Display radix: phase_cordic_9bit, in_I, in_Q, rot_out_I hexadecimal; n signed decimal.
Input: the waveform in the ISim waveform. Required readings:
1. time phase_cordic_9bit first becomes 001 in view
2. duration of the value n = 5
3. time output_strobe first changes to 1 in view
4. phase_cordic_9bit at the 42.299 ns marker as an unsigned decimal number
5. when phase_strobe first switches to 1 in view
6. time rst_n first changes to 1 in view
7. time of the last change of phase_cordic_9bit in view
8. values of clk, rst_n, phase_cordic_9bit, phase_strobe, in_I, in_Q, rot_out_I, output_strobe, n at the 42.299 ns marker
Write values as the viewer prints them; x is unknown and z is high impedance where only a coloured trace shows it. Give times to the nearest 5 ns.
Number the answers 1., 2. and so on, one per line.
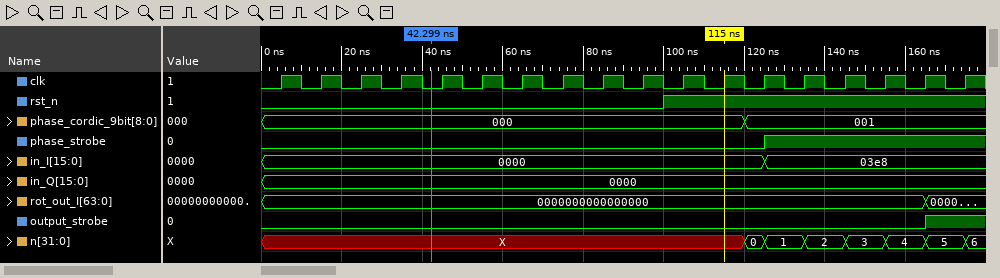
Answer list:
1. 120 ns
2. 10 ns
3. 165 ns
4. 0
5. 125 ns
6. 100 ns
7. 120 ns
8. clk=0, rst_n=0, phase_cordic_9bit=000, phase_strobe=0, in_I=0000, in_Q=0000, rot_out_I=0000000000000000, output_strobe=0, n=X
